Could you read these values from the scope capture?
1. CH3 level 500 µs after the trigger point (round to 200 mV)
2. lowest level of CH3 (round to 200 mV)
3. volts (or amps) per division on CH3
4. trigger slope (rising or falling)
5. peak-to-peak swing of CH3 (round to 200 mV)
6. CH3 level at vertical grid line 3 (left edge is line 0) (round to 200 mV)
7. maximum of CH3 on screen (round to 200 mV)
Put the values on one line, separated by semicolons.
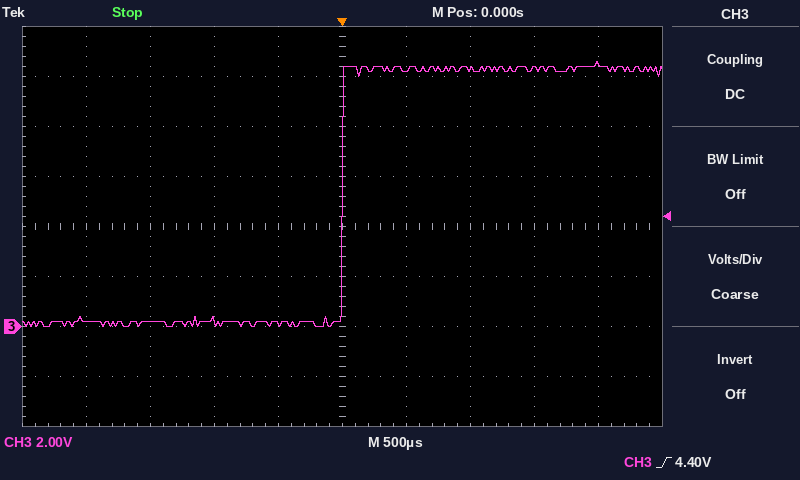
10.2 V; 0.0 V; 2 V; rising; 10.6 V; 200 mV; 10.6 V
